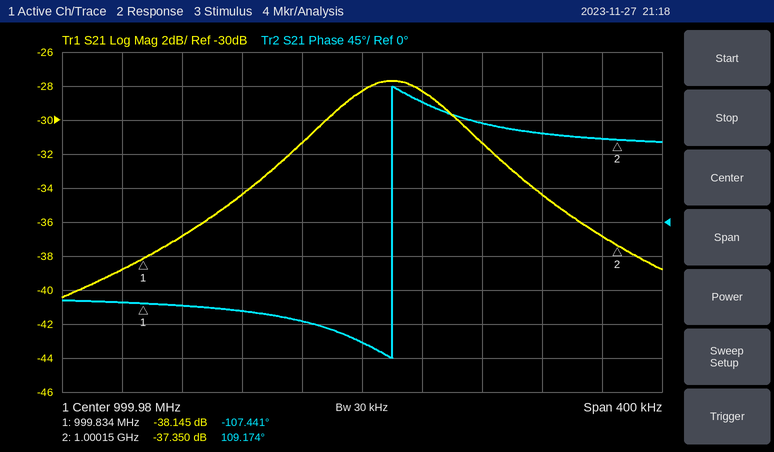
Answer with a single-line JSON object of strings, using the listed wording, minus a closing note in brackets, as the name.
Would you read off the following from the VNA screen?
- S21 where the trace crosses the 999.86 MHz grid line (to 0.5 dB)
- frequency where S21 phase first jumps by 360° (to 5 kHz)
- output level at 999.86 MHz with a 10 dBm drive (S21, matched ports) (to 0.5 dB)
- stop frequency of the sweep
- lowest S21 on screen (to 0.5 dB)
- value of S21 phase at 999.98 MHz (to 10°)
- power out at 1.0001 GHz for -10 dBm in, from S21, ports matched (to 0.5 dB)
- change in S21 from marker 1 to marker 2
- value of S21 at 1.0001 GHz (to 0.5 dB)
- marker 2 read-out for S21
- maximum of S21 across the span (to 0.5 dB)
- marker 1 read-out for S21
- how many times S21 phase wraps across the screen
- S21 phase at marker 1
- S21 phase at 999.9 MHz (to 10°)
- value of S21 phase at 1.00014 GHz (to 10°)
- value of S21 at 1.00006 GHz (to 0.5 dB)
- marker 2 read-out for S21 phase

{"S21 where the trace crosses the 999.86 MHz grid line": "-37.0 dB", "frequency where S21 phase first jumps by 360°": "1.000000 GHz", "output level at 999.86 MHz with a 10 dBm drive (S21, matched ports)": "-27.0 dBm", "stop frequency of the sweep": "1.00018 GHz", "lowest S21 on screen": "-40.5 dB", "value of S21 phase at 999.98 MHz": "-160°", "power out at 1.0001 GHz for -10 dBm in, from S21, ports matched": "-44.5 dBm", "change in S21 from marker 1 to marker 2": "0.795 dB", "value of S21 at 1.0001 GHz": "-34.5 dB", "marker 2 read-out for S21": "-37.350 dB", "maximum of S21 across the span": "-27.5 dB", "marker 1 read-out for S21": "-38.145 dB", "how many times S21 phase wraps across the screen": "1", "S21 phase at marker 1": "-107.441°", "S21 phase at 999.9 MHz": "-120°", "value of S21 phase at 1.00014 GHz": "110°", "value of S21 at 1.00006 GHz": "-31.5 dB", "marker 2 read-out for S21 phase": "109.174°"}
